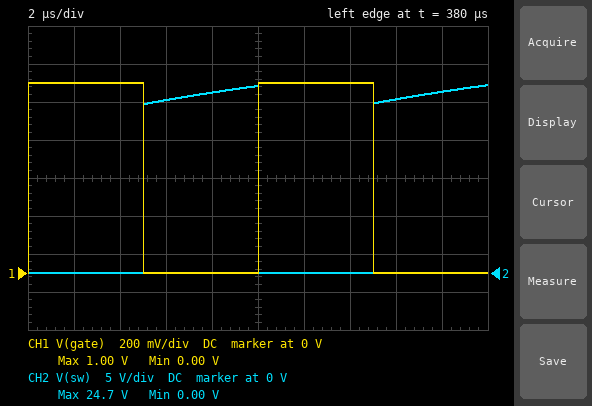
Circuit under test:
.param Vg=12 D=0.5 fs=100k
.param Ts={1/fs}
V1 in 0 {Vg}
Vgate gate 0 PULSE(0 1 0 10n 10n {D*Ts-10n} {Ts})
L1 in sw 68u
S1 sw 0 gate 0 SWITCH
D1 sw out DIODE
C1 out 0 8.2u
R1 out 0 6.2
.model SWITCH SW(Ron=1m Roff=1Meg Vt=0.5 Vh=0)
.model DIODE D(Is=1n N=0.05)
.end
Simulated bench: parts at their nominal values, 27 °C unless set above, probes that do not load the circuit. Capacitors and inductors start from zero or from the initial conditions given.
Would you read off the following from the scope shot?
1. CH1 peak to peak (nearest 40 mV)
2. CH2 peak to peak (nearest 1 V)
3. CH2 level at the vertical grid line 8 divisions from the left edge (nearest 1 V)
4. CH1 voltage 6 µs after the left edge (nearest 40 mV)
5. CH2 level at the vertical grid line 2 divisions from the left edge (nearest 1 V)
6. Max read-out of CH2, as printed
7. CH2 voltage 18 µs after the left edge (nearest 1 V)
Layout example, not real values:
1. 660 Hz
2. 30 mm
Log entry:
1. 1.00 V
2. 25 V
3. 23 V
4. 0 V
5. 0 V
6. 24.7 V
7. 24 V
